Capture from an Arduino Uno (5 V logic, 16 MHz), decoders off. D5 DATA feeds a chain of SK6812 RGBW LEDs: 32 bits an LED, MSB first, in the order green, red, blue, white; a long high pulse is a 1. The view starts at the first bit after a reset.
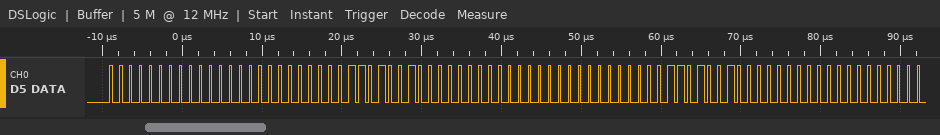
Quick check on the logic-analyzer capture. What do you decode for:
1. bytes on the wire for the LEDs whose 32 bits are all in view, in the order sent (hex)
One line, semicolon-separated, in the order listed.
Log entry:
00 00 00 D2 00 00 00 D2
